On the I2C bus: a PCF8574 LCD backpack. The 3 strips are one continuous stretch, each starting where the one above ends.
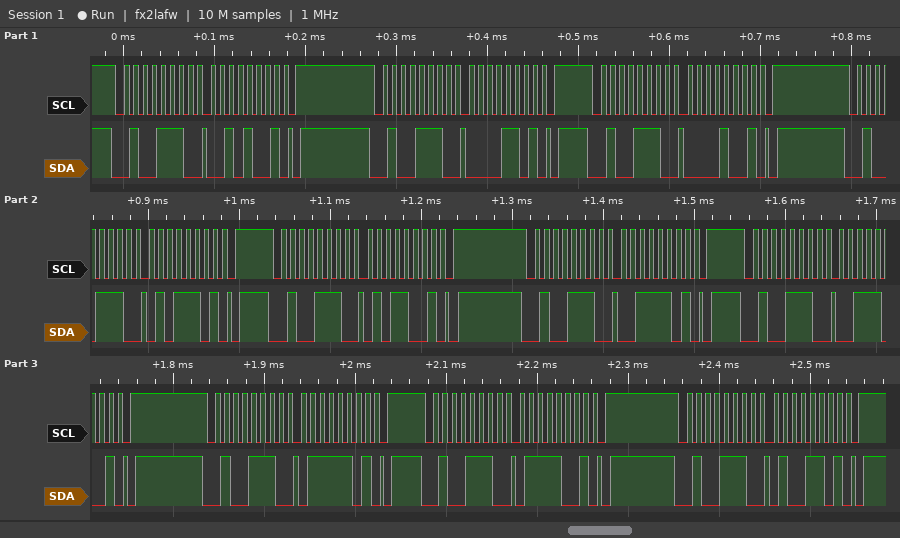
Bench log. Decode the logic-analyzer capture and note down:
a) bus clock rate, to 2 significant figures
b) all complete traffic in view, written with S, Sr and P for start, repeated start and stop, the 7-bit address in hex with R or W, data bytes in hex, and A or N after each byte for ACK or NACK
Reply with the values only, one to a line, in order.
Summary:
100 kHz
S 27W A 29 A P S 27W A 0D A P S 27W A 09 A P S 27W A 5D A P S 27W A 59 A P S 27W A 3D A P S 27W A 39 A P S 27W A 7D A P S 27W A 79 A P S 27W A 4D A P
